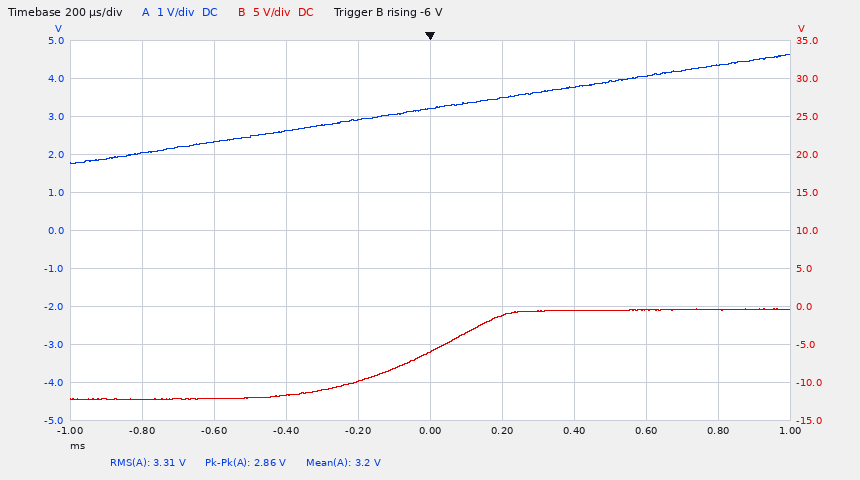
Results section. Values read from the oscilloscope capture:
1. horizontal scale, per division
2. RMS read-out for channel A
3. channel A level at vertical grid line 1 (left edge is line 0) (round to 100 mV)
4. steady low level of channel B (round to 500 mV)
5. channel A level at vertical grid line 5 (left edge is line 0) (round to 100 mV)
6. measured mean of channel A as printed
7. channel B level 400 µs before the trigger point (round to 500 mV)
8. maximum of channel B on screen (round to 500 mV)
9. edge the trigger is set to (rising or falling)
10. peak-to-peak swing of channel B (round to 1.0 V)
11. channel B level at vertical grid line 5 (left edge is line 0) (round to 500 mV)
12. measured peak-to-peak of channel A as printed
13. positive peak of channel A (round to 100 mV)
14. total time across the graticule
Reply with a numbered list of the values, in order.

1. 200 µs
2. 3.31 V
3. 2.0 V
4. -12.0 V
5. 3.2 V
6. 3.2 V
7. -11.5 V
8. -500 mV
9. rising
10. 12.0 V
11. -6.0 V
12. 2.86 V
13. 4.6 V
14. 2 ms
